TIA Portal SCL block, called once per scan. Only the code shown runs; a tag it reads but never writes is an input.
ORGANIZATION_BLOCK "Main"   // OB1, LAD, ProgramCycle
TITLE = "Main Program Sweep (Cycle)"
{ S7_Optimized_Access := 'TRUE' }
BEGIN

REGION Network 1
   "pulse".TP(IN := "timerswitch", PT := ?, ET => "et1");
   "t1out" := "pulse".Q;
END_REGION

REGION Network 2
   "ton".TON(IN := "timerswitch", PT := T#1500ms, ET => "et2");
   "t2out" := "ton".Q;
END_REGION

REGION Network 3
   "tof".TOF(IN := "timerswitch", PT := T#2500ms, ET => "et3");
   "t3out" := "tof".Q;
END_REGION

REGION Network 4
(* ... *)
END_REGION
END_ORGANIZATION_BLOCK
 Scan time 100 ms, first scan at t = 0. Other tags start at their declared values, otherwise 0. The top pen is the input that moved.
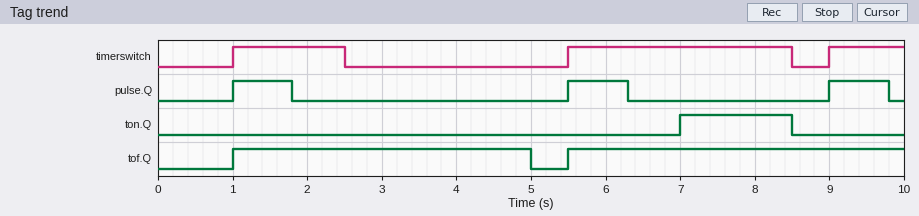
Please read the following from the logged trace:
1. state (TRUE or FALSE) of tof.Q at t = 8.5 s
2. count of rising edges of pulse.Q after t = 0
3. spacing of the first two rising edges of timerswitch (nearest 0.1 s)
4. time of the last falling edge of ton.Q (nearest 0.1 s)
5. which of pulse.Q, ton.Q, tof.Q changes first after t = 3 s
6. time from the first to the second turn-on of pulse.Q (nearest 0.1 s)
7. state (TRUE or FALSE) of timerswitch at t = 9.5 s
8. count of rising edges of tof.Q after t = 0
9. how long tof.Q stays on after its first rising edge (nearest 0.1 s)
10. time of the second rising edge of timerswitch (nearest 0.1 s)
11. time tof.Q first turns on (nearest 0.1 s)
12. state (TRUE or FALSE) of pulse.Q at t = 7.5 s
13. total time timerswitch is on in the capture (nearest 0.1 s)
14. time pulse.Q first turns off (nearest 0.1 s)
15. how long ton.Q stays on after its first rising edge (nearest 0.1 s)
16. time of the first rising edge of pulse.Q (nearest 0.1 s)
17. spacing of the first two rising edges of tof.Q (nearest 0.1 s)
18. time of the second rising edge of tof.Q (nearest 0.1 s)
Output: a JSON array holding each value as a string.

["TRUE", "3", "4.5 s", "8.5 s", "tof.Q", "4.5 s", "TRUE", "2", "4.0 s", "5.5 s", "1.0 s", "FALSE", "5.5 s", "1.8 s", "1.5 s", "1.0 s", "4.5 s", "5.5 s"]
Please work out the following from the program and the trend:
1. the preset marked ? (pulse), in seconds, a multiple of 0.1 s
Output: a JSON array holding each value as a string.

["0.8 s"]
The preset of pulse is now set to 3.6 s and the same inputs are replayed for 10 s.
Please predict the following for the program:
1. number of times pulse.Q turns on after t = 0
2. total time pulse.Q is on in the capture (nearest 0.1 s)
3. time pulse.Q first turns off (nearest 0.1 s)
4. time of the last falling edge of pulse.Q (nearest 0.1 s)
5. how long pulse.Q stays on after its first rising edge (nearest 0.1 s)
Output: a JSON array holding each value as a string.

["2", "7.2 s", "4.6 s", "9.1 s", "3.6 s"]
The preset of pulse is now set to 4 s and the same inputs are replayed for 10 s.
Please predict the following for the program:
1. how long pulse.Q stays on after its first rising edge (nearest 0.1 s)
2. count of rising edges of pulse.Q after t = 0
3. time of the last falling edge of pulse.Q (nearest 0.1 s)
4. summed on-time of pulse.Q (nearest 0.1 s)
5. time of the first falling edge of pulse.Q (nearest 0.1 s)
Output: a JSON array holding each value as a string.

["4.0 s", "2", "9.5 s", "8.0 s", "5.0 s"]
